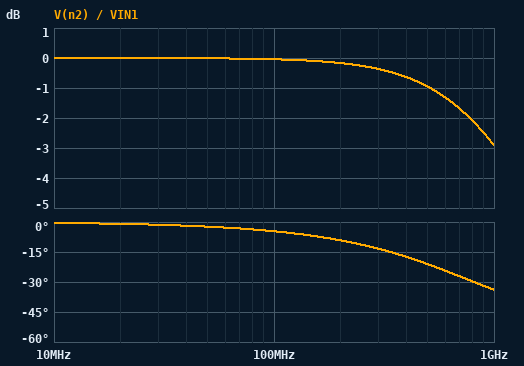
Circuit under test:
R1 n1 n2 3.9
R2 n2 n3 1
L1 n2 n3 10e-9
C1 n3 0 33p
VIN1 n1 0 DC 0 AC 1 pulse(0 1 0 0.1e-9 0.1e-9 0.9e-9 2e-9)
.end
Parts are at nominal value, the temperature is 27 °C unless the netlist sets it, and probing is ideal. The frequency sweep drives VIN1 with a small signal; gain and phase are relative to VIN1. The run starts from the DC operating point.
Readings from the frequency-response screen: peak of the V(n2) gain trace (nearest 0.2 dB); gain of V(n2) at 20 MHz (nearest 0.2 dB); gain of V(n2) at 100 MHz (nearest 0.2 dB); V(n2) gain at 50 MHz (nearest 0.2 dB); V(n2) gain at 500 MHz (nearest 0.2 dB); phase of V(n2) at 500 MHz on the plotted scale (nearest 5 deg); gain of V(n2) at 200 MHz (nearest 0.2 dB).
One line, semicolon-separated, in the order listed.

0 dB; 0 dB; 0 dB; 0 dB; -1.0 dB; -20 deg; -0.2 dB
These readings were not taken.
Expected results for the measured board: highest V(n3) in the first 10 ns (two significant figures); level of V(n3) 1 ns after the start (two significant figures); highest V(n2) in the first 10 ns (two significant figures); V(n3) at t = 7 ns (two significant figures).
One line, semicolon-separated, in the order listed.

1.0 V; 1.0 V; 1.0 V; 1.0 V
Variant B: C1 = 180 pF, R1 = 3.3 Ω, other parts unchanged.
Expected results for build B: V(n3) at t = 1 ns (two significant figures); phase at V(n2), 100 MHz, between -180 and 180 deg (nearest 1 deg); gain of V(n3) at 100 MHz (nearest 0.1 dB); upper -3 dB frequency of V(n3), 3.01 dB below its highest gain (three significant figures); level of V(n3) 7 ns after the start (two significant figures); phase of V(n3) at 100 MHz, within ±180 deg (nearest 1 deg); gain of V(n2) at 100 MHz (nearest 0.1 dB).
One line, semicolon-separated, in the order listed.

710 mV; -20 deg; -0.8 dB; 207 MHz; 780 mV; -26 deg; -0.9 dB
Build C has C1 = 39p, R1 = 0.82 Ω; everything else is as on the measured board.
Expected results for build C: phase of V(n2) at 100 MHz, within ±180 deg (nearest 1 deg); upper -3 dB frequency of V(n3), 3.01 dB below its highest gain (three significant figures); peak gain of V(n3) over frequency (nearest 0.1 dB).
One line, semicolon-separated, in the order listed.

-1 deg; 2.24 GHz; 0 dB
